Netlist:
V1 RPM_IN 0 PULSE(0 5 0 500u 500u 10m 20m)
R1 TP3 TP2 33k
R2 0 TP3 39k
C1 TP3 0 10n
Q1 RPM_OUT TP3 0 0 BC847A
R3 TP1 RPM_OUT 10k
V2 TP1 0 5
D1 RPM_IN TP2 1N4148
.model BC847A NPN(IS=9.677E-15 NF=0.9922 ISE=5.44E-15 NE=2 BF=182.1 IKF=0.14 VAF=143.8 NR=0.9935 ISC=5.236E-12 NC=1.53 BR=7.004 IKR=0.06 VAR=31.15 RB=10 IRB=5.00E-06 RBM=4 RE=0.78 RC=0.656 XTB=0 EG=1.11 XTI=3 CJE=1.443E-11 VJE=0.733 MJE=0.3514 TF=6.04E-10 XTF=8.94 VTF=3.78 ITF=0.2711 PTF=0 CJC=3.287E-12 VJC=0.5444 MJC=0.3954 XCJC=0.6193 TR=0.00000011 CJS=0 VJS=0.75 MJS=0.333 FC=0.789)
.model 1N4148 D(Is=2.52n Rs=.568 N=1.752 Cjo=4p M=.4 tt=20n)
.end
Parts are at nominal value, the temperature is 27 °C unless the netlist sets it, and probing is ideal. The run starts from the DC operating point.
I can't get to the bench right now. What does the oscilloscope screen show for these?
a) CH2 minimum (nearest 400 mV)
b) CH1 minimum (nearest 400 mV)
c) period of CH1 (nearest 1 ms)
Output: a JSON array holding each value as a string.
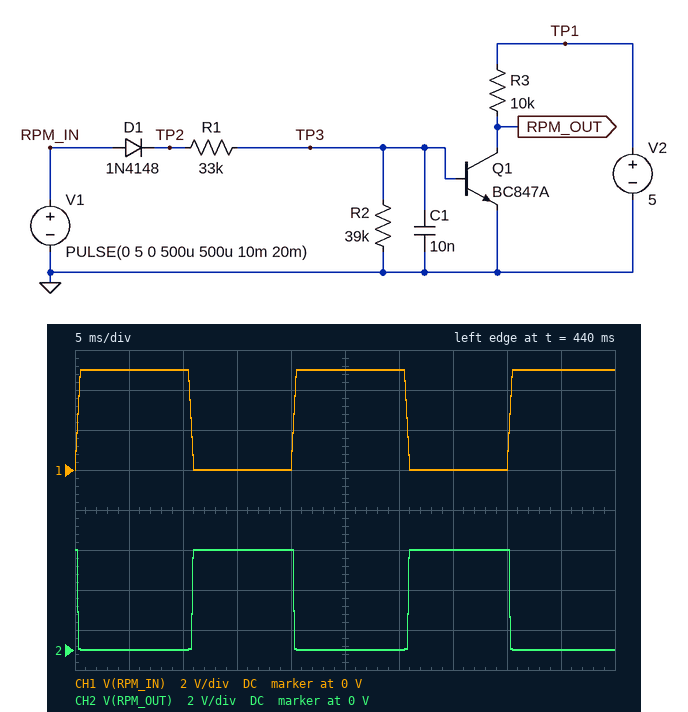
["0 V", "0 V", "20 ms"]
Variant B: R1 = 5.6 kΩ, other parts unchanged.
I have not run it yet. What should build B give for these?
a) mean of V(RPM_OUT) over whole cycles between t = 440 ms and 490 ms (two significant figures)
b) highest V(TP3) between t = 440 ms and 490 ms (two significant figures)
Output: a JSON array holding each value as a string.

["2.3 V", "690 mV"]
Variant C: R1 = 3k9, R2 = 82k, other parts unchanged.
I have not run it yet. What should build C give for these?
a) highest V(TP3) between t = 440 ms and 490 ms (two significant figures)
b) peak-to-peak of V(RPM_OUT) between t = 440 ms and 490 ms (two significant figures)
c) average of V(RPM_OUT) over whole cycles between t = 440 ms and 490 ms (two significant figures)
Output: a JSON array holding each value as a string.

["700 mV", "5.0 V", "2.3 V"]
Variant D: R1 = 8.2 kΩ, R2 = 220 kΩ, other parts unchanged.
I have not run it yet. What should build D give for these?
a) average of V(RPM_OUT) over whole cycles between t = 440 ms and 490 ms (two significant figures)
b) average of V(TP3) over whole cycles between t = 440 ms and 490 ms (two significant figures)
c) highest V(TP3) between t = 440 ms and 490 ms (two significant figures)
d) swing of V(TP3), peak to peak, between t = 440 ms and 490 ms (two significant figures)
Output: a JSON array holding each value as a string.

["2.3 V", "430 mV", "680 mV", "670 mV"]
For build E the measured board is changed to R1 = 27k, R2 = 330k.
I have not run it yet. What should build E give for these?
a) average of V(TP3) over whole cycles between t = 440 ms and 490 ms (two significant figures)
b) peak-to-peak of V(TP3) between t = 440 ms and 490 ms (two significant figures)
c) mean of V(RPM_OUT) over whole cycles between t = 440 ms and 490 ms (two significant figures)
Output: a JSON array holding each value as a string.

["450 mV", "620 mV", "2.3 V"]
